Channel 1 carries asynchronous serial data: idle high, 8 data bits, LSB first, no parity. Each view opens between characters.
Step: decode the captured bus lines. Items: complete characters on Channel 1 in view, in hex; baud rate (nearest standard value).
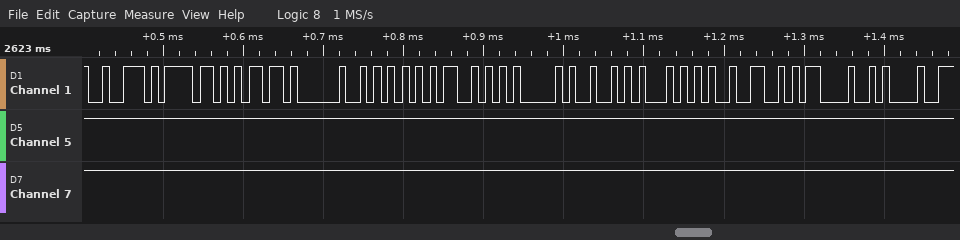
72, 6F, 6D, 20, 55, 53, 41, 52, 54, 32, 0D, 0A
115200 baud
